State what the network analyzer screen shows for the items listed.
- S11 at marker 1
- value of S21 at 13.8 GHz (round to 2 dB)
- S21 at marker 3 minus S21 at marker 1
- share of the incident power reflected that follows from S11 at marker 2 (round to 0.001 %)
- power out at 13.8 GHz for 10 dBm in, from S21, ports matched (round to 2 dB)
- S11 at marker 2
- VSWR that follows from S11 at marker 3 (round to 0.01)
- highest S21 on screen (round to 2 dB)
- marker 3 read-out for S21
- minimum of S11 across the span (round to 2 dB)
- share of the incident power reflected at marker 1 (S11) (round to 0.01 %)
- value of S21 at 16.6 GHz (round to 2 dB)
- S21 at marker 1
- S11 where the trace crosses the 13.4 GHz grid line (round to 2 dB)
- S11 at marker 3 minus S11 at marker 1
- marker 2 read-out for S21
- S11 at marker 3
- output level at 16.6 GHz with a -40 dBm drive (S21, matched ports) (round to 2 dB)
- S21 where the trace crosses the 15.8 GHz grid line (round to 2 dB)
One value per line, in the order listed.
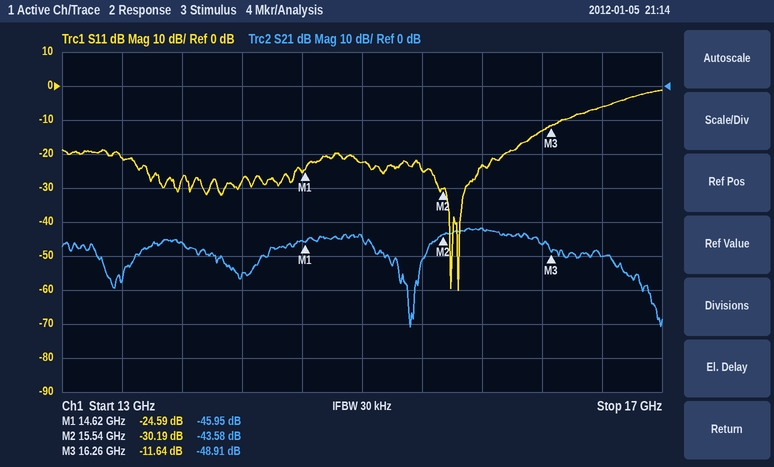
-24.59 dB
-46 dB
-2.96 dB
0.096 %
-36 dBm
-30.19 dB
1.71
-42 dB
-48.91 dB
-60 dB
0.35 %
-50 dB
-45.95 dB
-22 dB
12.95 dB
-43.58 dB
-11.64 dB
-90 dBm
-42 dB
